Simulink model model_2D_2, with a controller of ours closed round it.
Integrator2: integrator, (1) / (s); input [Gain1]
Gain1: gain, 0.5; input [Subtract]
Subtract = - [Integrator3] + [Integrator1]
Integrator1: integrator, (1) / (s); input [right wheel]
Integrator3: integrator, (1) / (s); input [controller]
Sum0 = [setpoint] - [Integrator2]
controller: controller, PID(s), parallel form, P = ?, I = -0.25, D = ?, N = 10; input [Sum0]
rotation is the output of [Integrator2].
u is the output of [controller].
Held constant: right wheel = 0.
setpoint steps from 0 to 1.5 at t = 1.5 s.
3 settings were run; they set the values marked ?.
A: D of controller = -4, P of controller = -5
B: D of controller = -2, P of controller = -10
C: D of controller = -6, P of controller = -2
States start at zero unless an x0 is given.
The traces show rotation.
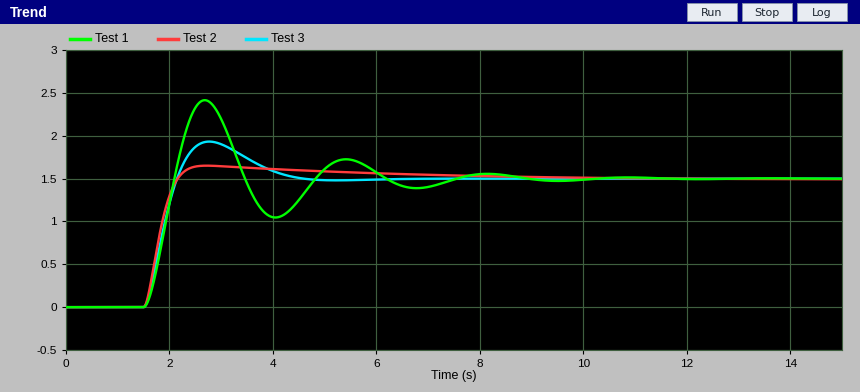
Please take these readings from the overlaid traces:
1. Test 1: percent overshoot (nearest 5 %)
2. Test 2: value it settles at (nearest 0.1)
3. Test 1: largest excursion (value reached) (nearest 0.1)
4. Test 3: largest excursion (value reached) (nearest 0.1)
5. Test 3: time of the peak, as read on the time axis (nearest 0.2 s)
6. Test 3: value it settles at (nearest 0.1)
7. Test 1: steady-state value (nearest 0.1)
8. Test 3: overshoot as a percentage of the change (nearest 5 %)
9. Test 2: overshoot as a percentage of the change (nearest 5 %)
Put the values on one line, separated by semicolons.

60 %; 1.5; 2.4; 1.9; 2.8 s; 1.5; 1.5; 30 %; 10 %
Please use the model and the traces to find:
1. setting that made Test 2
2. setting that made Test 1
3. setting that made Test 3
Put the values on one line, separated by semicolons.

C; B; A
